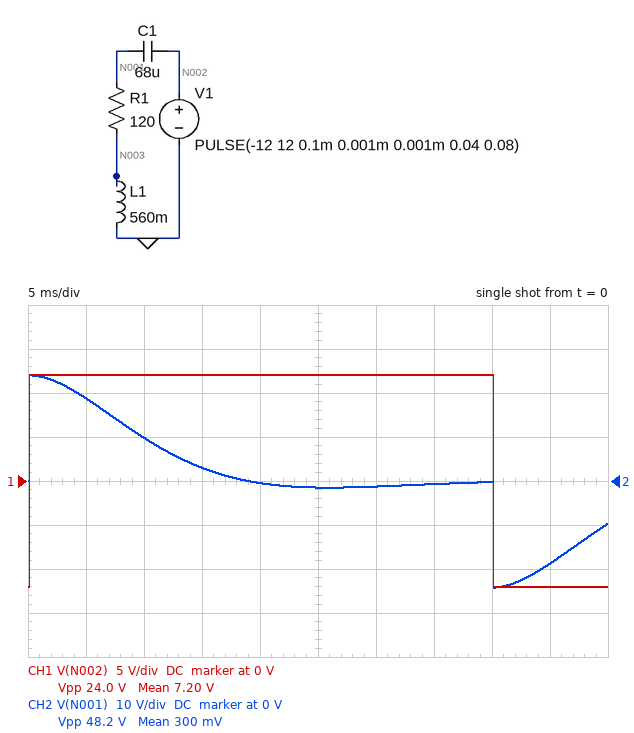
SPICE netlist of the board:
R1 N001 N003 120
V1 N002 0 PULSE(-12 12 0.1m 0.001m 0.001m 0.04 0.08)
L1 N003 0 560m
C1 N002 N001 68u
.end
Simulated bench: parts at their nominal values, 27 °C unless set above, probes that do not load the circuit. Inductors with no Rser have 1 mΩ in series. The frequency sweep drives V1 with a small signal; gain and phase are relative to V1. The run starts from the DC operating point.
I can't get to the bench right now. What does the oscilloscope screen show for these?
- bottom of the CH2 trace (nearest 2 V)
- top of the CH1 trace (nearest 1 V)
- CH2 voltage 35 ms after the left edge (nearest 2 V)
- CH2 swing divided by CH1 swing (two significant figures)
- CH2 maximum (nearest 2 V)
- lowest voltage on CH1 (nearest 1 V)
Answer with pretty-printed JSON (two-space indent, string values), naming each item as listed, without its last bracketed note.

{
  "bottom of the CH2 trace": "-24 V",
  "top of the CH1 trace": "12 V",
  "CH2 voltage 35 ms after the left edge": "0 V",
  "CH2 swing divided by CH1 swing": "2.0",
  "CH2 maximum": "24 V",
  "lowest voltage on CH1": "-12 V"
}
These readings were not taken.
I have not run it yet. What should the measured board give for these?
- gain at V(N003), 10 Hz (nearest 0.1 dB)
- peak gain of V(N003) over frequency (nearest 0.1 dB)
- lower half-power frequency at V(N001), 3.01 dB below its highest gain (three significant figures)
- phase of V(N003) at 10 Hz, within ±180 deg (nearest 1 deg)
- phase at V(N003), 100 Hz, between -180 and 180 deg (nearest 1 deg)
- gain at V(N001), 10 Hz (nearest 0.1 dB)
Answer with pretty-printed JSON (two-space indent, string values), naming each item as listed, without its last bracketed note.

{
  "gain at V(N003), 10 Hz": "-16.4 dB",
  "peak gain of V(N003) over frequency": "0.1 dB",
  "lower half-power frequency at V(N001), 3.01 dB below its highest gain": "16.7 Hz",
  "phase of V(N003) at 10 Hz, within ±180 deg": "149 deg",
  "phase at V(N003), 100 Hz, between -180 and 180 deg": "20 deg",
  "gain at V(N001), 10 Hz": "-5.4 dB"
}
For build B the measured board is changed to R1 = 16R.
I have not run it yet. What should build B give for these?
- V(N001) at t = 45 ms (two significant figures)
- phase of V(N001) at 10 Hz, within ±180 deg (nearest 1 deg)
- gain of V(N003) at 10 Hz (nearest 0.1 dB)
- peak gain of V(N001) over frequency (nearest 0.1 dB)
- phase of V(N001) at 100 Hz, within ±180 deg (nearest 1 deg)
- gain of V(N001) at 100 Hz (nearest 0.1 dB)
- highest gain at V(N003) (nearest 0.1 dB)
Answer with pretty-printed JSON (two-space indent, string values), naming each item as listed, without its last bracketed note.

{
  "V(N001) at t = 45 ms": "-9.0 V",
  "phase of V(N001) at 10 Hz, within ±180 deg": "151 deg",
  "gain of V(N003) at 10 Hz": "-15.1 dB",
  "peak gain of V(N001) over frequency": "15.2 dB",
  "phase of V(N001) at 100 Hz, within ±180 deg": "0 deg",
  "gain of V(N001) at 100 Hz": "0.6 dB",
  "highest gain at V(N003)": "15.1 dB"
}
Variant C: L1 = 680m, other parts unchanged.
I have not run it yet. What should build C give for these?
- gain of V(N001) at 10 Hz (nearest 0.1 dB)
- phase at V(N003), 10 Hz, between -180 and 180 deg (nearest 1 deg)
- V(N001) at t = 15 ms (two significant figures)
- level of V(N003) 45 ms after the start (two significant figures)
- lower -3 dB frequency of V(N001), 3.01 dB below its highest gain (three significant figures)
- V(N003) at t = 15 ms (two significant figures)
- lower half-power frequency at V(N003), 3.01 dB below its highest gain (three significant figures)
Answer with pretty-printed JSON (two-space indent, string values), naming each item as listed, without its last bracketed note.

{
  "gain of V(N001) at 10 Hz": "-5.0 dB",
  "phase at V(N003), 10 Hz, between -180 and 180 deg": "148 deg",
  "V(N001) at t = 15 ms": "3.6 V",
  "level of V(N003) 45 ms after the start": "-6.2 V",
  "lower -3 dB frequency of V(N001), 3.01 dB below its highest gain": "15.9 Hz",
  "V(N003) at t = 15 ms": "-5.9 V",
  "lower half-power frequency at V(N003), 3.01 dB below its highest gain": "21.0 Hz"
}
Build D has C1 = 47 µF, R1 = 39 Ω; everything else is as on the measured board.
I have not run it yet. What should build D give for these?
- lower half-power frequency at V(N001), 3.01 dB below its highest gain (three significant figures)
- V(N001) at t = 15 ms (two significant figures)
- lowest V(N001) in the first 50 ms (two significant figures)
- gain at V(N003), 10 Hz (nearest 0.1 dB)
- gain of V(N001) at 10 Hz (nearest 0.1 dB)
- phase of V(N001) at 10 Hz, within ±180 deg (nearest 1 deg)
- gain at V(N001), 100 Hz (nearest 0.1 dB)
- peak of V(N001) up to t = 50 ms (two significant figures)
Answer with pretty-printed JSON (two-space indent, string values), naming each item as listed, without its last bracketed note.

{
  "lower half-power frequency at V(N001), 3.01 dB below its highest gain": "27.2 Hz",
  "V(N001) at t = 15 ms": "-13 V",
  "lowest V(N001) in the first 50 ms": "-23 V",
  "gain at V(N003), 10 Hz": "-18.8 dB",
  "gain of V(N001) at 10 Hz": "-15.3 dB",
  "phase of V(N001) at 10 Hz, within ±180 deg": "125 deg",
  "gain at V(N001), 100 Hz": "0.9 dB",
  "peak of V(N001) up to t = 50 ms": "24 V"
}
